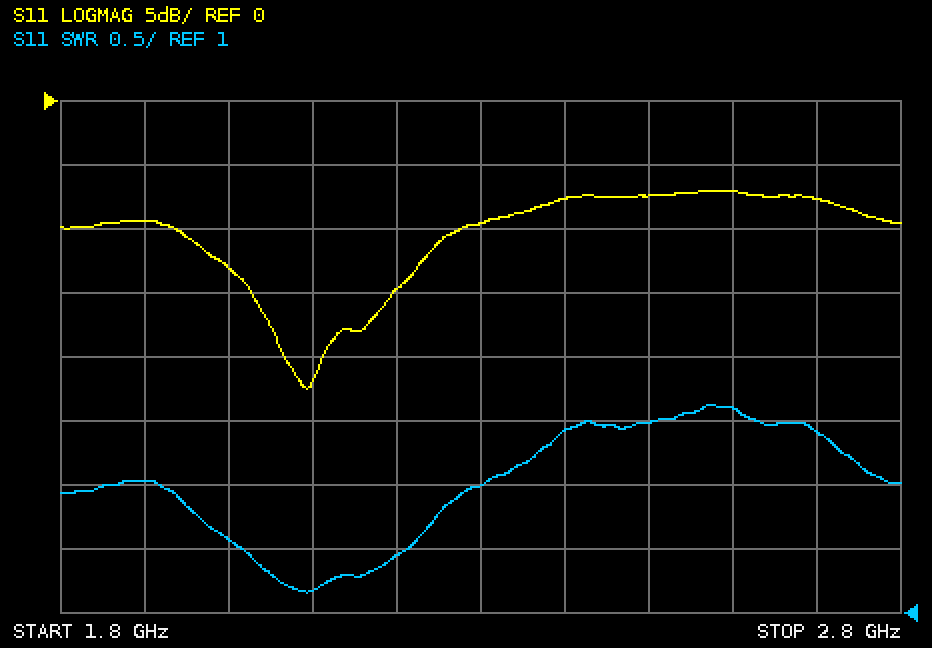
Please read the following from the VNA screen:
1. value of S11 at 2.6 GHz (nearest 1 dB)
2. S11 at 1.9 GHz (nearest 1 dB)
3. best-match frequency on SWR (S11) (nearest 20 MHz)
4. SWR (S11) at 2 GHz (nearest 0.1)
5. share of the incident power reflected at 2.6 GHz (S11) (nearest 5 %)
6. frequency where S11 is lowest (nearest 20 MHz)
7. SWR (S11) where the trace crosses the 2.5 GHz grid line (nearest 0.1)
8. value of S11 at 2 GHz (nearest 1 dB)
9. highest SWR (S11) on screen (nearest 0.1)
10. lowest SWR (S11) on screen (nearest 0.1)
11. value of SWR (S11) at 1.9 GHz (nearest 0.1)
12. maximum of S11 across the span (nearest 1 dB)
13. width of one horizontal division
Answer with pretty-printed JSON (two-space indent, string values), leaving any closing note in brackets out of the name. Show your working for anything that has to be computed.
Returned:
{
  "value of S11 at 2.6 GHz": "-7 dB",
  "S11 at 1.9 GHz": "-9 dB",
  "best-match frequency on SWR (S11)": "2.10 GHz",
  "SWR (S11) at 2 GHz": "1.6",
  "share of the incident power reflected at 2.6 GHz (S11)": "10^(-7/10) ≈ 20 %",
  "frequency where S11 is lowest": "2.10 GHz",
  "SWR (S11) where the trace crosses the 2.5 GHz grid line": "2.5",
  "value of S11 at 2 GHz": "-13 dB",
  "highest SWR (S11) on screen": "2.6",
  "lowest SWR (S11) on screen": "1.2",
  "value of SWR (S11) at 1.9 GHz": "2.0",
  "maximum of S11 across the span": "-7 dB",
  "width of one horizontal division": "100 MHz"
}
